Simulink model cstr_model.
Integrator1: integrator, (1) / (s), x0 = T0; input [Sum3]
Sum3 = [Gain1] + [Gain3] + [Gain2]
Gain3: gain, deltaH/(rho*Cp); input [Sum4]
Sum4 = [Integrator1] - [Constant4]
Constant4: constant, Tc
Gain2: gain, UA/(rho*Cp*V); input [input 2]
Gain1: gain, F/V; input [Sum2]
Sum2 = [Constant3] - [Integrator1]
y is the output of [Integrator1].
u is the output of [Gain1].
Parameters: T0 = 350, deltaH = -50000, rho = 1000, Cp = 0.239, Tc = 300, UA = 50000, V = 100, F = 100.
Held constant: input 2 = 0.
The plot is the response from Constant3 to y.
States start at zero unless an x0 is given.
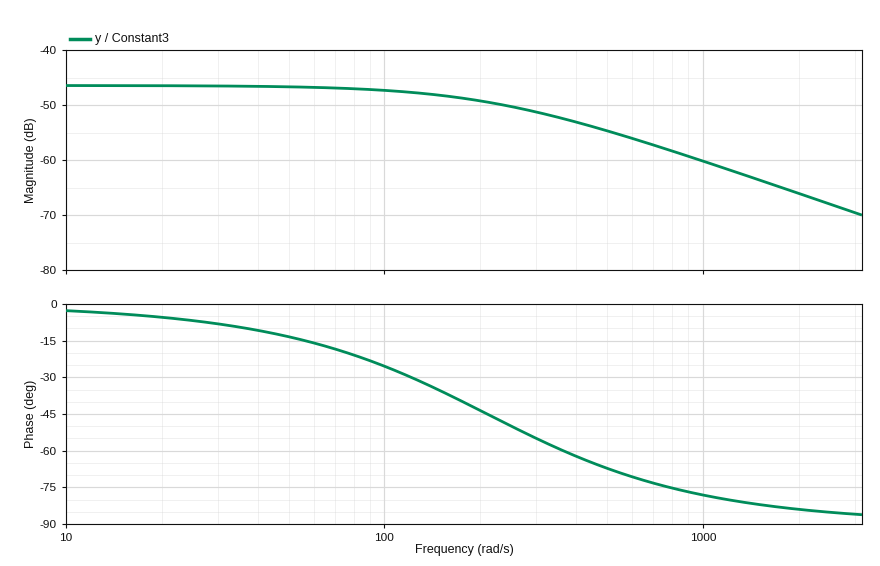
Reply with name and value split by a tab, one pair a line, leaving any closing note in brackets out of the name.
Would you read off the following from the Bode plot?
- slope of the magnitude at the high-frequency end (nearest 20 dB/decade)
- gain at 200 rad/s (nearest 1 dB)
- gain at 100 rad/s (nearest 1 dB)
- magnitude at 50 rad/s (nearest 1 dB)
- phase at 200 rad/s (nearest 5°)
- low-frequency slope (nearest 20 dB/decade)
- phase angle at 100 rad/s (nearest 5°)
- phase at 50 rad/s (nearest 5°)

slope of the magnitude at the high-frequency end	-20 dB/decade
gain at 200 rad/s	-49 dB
gain at 100 rad/s	-47 dB
magnitude at 50 rad/s	-47 dB
phase at 200 rad/s	-45°
low-frequency slope	0 dB/decade
phase angle at 100 rad/s	-25°
phase at 50 rad/s	-15°
